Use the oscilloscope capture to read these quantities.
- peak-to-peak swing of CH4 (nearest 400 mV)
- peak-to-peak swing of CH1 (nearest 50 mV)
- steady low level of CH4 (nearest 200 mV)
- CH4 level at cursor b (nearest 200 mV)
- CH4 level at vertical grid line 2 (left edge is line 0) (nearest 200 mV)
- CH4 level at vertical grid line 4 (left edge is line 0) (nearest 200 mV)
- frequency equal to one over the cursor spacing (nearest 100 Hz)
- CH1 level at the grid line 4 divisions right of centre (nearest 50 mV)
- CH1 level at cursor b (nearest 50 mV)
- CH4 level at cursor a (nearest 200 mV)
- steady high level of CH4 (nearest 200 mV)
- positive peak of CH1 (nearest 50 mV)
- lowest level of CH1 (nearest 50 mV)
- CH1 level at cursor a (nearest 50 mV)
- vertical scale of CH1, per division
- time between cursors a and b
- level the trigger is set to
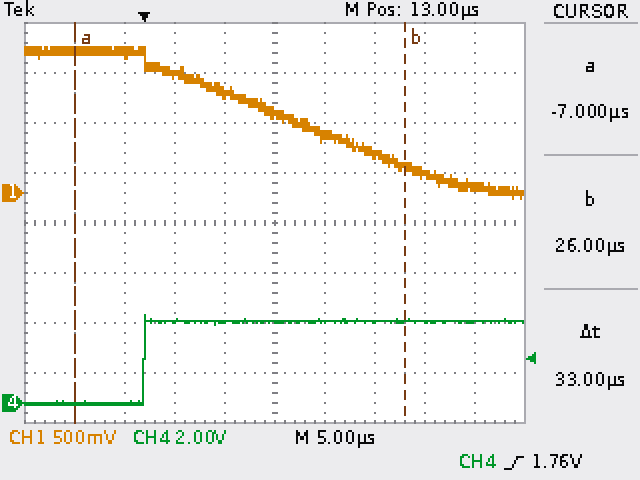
3.6 V
1.50 V
0.0 V
3.2 V
0.0 V
3.2 V
30.3 kHz
50 mV
250 mV
0.0 V
3.2 V
1.45 V
-50 mV
1.40 V
500 mV
33 µs
1.76 V
